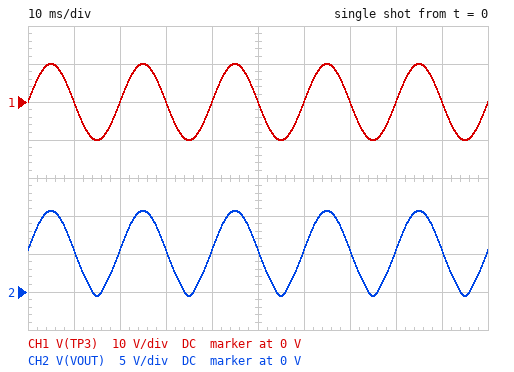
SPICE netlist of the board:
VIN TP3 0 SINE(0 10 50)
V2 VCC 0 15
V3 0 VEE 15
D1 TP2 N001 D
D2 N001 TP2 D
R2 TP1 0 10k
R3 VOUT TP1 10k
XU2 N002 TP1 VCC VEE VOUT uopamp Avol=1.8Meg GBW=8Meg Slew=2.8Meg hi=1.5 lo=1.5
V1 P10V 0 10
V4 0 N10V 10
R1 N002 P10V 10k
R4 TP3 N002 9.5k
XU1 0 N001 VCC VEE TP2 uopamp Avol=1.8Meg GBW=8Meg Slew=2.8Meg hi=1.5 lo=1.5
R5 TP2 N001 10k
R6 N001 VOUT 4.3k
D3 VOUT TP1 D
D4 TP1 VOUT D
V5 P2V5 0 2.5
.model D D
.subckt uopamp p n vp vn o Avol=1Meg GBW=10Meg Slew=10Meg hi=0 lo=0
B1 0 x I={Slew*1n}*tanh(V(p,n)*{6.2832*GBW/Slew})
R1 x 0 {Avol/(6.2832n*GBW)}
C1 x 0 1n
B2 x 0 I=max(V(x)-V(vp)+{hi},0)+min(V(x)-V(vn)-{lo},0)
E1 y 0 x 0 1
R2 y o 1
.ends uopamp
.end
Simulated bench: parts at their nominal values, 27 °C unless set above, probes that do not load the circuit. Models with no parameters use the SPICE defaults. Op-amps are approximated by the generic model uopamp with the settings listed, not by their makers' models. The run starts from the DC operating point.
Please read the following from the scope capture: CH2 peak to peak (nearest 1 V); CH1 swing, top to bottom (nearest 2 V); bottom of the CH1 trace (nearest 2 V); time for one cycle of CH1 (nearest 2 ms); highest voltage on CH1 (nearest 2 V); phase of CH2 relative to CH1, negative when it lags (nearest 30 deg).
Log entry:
11 V
20 V
-10 V
20 ms
10 V
0 deg
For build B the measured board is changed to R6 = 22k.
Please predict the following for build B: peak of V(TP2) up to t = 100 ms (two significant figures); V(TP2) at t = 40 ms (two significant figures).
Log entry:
230 mV
-610 mV
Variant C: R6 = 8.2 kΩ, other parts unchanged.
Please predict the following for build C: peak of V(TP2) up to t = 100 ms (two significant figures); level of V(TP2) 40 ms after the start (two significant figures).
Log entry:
530 mV
-640 mV
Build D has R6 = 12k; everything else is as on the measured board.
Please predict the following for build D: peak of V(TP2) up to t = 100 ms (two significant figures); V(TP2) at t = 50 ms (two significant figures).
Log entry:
430 mV
-630 mV
